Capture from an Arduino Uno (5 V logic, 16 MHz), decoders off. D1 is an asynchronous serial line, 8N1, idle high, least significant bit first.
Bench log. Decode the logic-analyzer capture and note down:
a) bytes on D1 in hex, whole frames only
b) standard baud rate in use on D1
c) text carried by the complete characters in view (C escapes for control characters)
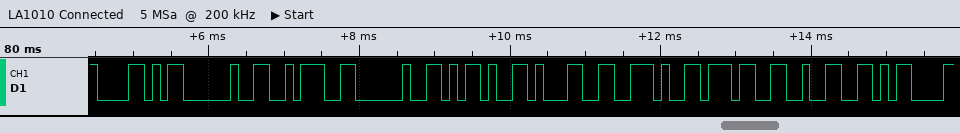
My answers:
0x58 0x20 0x3A 0x20 0x2D 0x31 0x2E 0x37 0x32 0x0D
9600 baud
"X : -1.72\r"
